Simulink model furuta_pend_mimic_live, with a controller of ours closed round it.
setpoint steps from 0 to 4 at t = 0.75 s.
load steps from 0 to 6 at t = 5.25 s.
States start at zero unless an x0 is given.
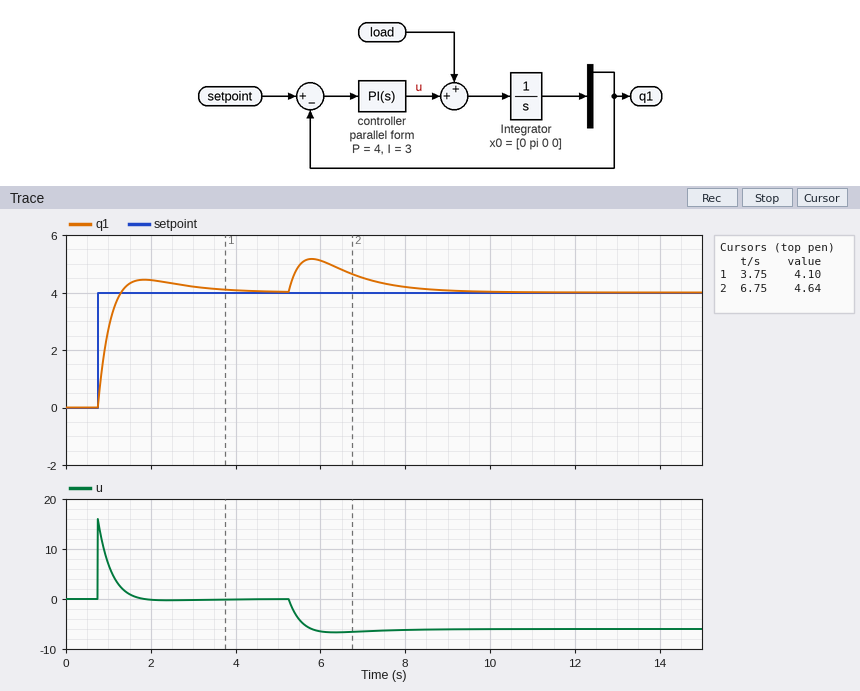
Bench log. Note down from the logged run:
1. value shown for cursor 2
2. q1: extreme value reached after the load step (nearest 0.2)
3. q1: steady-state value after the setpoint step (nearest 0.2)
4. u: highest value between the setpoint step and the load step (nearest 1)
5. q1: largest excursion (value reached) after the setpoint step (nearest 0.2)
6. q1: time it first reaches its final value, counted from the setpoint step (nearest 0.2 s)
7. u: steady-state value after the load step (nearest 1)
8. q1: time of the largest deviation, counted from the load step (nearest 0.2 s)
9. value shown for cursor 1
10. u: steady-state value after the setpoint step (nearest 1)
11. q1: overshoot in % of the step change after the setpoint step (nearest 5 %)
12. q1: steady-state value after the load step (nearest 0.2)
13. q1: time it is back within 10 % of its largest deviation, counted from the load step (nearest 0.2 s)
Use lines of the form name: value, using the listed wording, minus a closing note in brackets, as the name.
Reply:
value shown for cursor 2: 4.64
q1: extreme value reached after the load step: 5.2
q1: steady-state value after the setpoint step: 4.0
u: highest value between the setpoint step and the load step: 16
q1: largest excursion (value reached) after the setpoint step: 4.4
q1: time it first reaches its final value, counted from the setpoint step: 0.6 s
u: steady-state value after the load step: -6
q1: time of the largest deviation, counted from the load step: 0.6 s
value shown for cursor 1: 4.10
u: steady-state value after the setpoint step: 0
q1: overshoot in % of the step change after the setpoint step: 10 %
q1: steady-state value after the load step: 4.0
q1: time it is back within 10 % of its largest deviation, counted from the load step: 3.2 s
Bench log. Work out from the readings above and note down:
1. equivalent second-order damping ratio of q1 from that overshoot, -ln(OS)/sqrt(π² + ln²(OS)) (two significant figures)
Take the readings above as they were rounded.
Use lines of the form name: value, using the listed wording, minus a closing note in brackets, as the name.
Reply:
equivalent second-order damping ratio of q1 from that overshoot, -ln(OS)/sqrt(π² + ln²(OS)): 0.59
